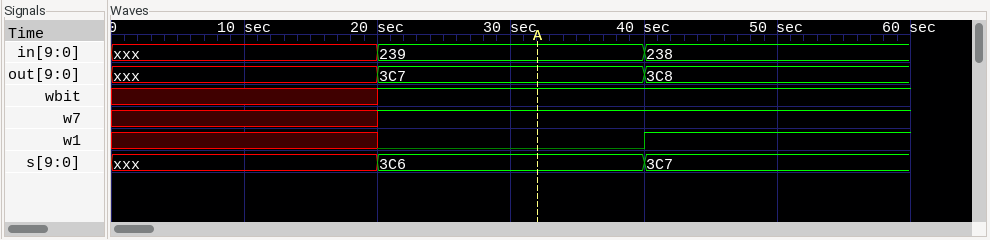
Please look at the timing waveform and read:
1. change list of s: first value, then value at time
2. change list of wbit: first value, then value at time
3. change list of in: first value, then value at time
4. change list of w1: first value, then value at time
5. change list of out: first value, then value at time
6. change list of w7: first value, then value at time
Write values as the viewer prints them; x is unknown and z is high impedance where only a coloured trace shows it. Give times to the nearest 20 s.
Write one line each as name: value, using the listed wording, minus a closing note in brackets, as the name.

change list of s: first value, then value at time: xxx, 3C6 at 20 s, 3C7 at 40 s
change list of wbit: first value, then value at time: x, 1 at 20 s
change list of in: first value, then value at time: xxx, 239 at 20 s, 238 at 40 s
change list of w1: first value, then value at time: x, 0 at 20 s, 1 at 40 s
change list of out: first value, then value at time: xxx, 3C7 at 20 s, 3C8 at 40 s
change list of w7: first value, then value at time: x, 1 at 20 s
